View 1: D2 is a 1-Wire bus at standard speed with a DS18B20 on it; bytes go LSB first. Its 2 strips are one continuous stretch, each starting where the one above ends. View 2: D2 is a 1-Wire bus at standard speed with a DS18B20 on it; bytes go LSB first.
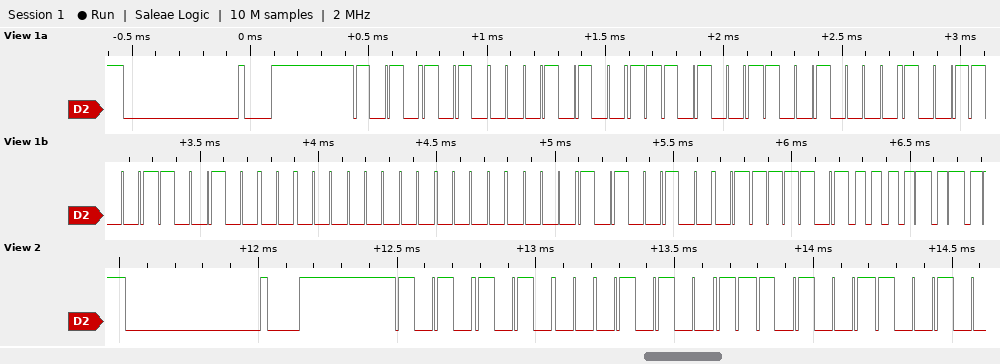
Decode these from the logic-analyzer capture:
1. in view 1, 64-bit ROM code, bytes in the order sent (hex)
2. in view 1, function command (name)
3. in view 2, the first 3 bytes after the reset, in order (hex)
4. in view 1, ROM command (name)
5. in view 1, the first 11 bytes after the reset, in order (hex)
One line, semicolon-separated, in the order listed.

28 97 09 99 09 00 00 25; Read Scratchpad; 55 28 97; Match ROM; 55 28 97 09 99 09 00 00 25 BE 50
